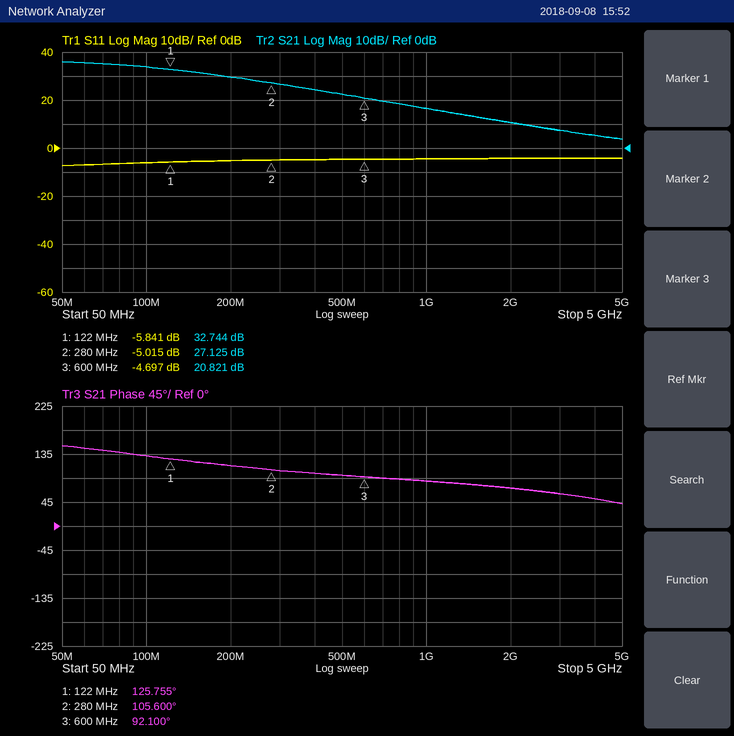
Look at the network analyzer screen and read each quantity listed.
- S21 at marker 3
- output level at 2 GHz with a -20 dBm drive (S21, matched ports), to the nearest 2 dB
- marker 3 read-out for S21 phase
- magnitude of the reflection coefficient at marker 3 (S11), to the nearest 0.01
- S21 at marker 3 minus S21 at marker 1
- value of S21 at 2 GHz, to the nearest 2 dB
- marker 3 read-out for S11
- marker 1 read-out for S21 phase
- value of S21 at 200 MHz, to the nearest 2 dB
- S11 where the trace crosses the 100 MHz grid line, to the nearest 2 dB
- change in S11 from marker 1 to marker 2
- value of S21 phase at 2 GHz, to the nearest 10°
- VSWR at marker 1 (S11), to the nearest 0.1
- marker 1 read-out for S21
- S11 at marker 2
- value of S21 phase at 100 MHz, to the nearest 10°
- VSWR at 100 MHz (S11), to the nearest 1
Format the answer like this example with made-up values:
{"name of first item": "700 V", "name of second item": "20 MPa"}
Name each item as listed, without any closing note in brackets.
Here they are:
{"S21 at marker 3": "20.821 dB", "output level at 2 GHz with a -20 dBm drive (S21, matched ports), to the nearest 2 dB": "-10 dBm", "marker 3 read-out for S21 phase": "92.100°", "magnitude of the reflection coefficient at marker 3 (S11), to the nearest 0.01": "0.58", "S21 at marker 3 minus S21 at marker 1": "-11.923 dB", "value of S21 at 2 GHz, to the nearest 2 dB": "10 dB", "marker 3 read-out for S11": "-4.697 dB", "marker 1 read-out for S21 phase": "125.755°", "value of S21 at 200 MHz, to the nearest 2 dB": "30 dB", "S11 where the trace crosses the 100 MHz grid line, to the nearest 2 dB": "-6 dB", "change in S11 from marker 1 to marker 2": "0.826 dB", "value of S21 phase at 2 GHz, to the nearest 10°": "70°", "VSWR at marker 1 (S11), to the nearest 0.1": "3.1", "marker 1 read-out for S21": "32.744 dB", "S11 at marker 2": "-5.015 dB", "value of S21 phase at 100 MHz, to the nearest 10°": "130°", "VSWR at 100 MHz (S11), to the nearest 1": "3"}
